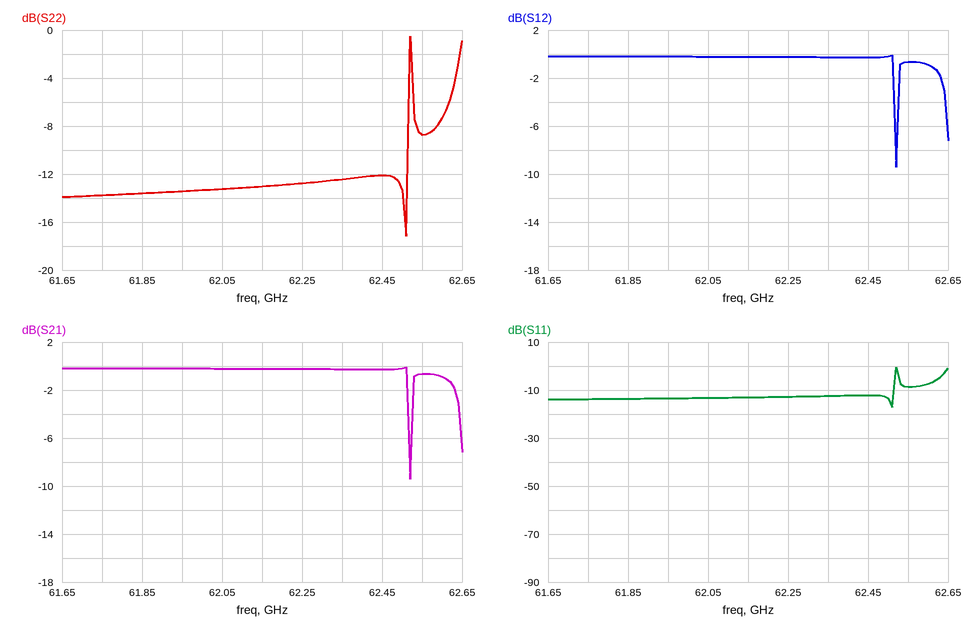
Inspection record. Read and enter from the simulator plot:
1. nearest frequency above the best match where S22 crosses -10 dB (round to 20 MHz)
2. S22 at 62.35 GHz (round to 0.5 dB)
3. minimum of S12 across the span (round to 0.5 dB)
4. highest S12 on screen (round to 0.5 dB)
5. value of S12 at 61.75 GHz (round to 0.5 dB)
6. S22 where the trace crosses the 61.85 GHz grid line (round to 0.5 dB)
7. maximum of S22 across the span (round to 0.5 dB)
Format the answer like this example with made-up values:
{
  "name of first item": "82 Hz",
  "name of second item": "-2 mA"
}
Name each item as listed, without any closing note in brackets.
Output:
{
  "nearest frequency above the best match where S22 crosses -10 dB": "62.52 GHz",
  "S22 at 62.35 GHz": "-12.5 dB",
  "minimum of S12 across the span": "-9.5 dB",
  "highest S12 on screen": "0.0 dB",
  "value of S12 at 61.75 GHz": "0.0 dB",
  "S22 where the trace crosses the 61.85 GHz grid line": "-13.5 dB",
  "maximum of S22 across the span": "-0.5 dB"
}
